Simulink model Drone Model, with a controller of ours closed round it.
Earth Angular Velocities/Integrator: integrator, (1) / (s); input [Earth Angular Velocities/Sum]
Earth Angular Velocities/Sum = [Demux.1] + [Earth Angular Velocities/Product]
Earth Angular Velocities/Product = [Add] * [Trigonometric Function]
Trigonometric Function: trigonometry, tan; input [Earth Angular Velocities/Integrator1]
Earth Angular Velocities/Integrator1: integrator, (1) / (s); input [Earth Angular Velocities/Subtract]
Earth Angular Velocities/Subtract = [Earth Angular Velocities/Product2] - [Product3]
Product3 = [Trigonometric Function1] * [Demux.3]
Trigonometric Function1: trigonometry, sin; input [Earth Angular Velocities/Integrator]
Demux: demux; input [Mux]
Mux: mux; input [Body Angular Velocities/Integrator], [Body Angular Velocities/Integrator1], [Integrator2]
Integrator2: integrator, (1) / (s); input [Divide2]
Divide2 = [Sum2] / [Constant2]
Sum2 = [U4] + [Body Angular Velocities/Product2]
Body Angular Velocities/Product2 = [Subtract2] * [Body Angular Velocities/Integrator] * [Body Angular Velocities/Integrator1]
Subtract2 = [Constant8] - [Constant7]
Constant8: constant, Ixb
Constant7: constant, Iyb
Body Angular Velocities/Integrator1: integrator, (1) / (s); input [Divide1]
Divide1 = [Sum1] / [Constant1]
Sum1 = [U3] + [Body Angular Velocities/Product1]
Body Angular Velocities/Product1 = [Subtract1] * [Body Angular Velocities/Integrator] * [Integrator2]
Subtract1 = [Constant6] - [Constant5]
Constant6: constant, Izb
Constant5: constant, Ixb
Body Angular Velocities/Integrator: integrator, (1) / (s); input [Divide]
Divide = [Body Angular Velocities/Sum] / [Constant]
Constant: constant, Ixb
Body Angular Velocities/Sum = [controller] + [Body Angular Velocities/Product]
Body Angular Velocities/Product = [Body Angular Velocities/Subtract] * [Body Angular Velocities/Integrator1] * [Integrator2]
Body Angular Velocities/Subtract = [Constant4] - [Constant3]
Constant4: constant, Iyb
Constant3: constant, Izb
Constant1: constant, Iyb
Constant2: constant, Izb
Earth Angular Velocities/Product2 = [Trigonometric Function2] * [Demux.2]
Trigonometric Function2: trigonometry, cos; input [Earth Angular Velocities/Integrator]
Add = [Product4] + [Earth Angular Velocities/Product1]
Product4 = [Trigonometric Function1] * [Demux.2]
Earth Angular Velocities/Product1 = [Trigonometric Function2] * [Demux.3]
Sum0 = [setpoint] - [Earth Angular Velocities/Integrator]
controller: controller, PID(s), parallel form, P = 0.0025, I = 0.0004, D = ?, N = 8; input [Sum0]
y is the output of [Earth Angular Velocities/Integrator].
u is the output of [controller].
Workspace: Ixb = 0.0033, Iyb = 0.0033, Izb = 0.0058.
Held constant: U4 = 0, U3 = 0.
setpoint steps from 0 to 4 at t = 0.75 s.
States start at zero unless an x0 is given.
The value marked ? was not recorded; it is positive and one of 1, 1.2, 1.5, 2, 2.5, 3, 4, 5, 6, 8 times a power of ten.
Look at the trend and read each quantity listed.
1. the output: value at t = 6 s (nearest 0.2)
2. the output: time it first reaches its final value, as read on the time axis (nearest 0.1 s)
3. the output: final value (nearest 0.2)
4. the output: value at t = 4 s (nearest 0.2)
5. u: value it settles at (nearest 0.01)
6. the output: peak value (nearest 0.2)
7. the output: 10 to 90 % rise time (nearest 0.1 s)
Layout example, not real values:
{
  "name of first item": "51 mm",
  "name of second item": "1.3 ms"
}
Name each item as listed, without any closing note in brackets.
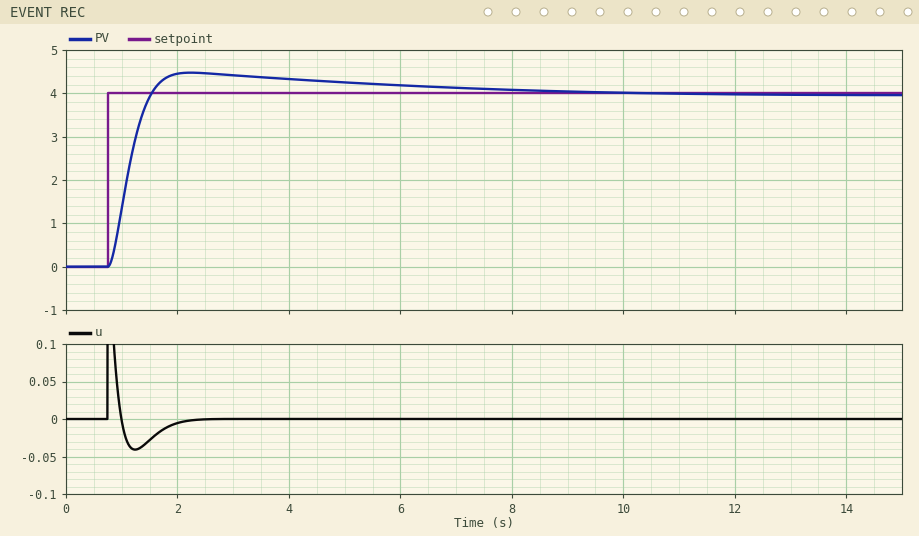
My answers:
{
  "the output: value at t = 6 s": "4.2",
  "the output: time it first reaches its final value, as read on the time axis": "1.5 s",
  "the output: final value": "4.0",
  "the output: value at t = 4 s": "4.4",
  "u: value it settles at": "0.00",
  "the output: peak value": "4.4",
  "the output: 10 to 90 % rise time": "0.5 s"
}
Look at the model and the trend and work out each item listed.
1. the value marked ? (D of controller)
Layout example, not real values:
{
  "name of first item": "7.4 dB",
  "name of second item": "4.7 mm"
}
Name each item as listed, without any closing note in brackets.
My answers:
{
  "the value marked ?": "0.008"
}
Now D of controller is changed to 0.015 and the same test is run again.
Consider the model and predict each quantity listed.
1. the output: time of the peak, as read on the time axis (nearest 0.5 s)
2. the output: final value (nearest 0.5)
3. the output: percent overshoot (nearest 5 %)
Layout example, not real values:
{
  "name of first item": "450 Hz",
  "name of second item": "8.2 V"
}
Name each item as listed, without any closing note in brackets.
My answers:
{
  "the output: time of the peak, as read on the time axis": "1.5 s",
  "the output: final value": "4.0",
  "the output: percent overshoot": "10 %"
}
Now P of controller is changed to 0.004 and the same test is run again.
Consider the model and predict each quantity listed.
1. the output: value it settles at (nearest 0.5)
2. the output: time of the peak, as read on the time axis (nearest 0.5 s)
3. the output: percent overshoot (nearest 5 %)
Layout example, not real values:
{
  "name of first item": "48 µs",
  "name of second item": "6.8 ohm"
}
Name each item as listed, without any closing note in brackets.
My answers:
{
  "the output: value it settles at": "4.0",
  "the output: time of the peak, as read on the time axis": "2.0 s",
  "the output: percent overshoot": "15 %"
}
